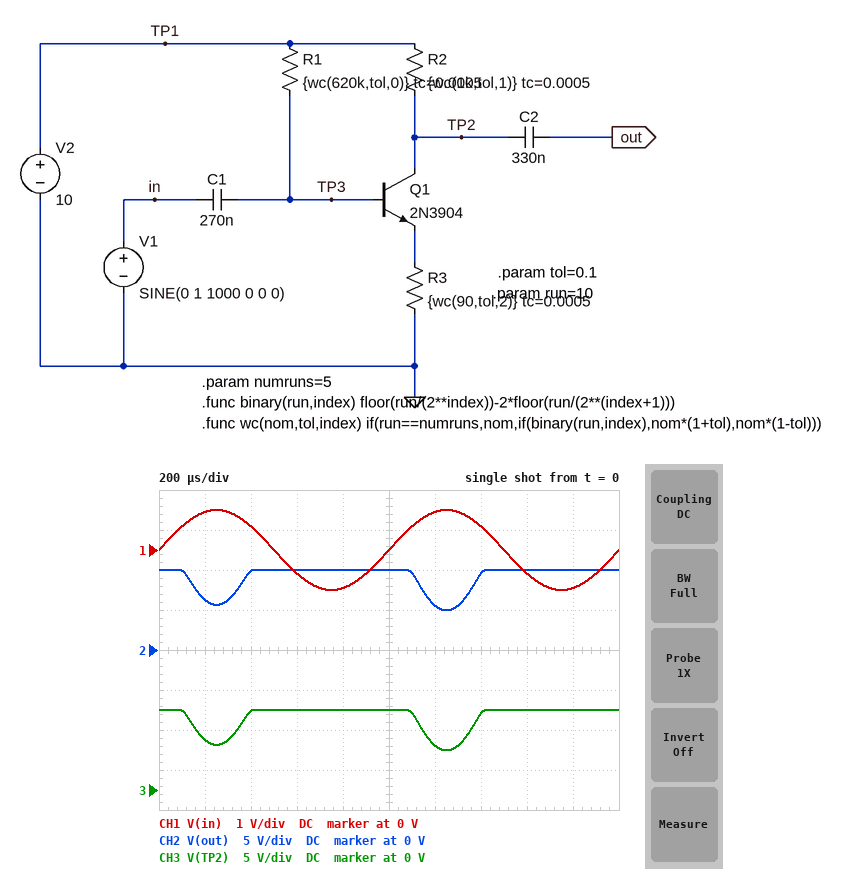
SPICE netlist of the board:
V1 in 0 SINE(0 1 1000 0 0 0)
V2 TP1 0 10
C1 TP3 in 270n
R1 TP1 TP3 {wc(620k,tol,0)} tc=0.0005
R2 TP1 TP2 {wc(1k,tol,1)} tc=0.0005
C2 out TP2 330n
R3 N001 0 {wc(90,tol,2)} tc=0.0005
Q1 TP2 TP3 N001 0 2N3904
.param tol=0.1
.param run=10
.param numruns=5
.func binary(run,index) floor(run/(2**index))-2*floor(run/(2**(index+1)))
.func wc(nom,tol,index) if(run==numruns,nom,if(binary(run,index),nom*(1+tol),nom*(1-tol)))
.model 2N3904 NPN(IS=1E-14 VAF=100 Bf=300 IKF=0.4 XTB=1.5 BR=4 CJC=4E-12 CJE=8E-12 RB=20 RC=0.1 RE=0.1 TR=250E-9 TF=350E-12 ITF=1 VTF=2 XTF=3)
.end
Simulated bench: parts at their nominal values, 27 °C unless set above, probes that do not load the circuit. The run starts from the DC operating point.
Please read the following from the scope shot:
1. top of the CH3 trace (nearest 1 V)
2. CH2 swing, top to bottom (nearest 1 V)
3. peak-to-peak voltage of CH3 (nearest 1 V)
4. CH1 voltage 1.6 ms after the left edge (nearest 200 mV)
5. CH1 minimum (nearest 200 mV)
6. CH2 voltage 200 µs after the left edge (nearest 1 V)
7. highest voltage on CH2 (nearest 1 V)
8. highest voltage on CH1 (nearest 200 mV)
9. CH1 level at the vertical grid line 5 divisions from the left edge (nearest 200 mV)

10 V
5 V
5 V
-600 mV
-1.0 V
6 V
10 V
1.0 V
0 V
